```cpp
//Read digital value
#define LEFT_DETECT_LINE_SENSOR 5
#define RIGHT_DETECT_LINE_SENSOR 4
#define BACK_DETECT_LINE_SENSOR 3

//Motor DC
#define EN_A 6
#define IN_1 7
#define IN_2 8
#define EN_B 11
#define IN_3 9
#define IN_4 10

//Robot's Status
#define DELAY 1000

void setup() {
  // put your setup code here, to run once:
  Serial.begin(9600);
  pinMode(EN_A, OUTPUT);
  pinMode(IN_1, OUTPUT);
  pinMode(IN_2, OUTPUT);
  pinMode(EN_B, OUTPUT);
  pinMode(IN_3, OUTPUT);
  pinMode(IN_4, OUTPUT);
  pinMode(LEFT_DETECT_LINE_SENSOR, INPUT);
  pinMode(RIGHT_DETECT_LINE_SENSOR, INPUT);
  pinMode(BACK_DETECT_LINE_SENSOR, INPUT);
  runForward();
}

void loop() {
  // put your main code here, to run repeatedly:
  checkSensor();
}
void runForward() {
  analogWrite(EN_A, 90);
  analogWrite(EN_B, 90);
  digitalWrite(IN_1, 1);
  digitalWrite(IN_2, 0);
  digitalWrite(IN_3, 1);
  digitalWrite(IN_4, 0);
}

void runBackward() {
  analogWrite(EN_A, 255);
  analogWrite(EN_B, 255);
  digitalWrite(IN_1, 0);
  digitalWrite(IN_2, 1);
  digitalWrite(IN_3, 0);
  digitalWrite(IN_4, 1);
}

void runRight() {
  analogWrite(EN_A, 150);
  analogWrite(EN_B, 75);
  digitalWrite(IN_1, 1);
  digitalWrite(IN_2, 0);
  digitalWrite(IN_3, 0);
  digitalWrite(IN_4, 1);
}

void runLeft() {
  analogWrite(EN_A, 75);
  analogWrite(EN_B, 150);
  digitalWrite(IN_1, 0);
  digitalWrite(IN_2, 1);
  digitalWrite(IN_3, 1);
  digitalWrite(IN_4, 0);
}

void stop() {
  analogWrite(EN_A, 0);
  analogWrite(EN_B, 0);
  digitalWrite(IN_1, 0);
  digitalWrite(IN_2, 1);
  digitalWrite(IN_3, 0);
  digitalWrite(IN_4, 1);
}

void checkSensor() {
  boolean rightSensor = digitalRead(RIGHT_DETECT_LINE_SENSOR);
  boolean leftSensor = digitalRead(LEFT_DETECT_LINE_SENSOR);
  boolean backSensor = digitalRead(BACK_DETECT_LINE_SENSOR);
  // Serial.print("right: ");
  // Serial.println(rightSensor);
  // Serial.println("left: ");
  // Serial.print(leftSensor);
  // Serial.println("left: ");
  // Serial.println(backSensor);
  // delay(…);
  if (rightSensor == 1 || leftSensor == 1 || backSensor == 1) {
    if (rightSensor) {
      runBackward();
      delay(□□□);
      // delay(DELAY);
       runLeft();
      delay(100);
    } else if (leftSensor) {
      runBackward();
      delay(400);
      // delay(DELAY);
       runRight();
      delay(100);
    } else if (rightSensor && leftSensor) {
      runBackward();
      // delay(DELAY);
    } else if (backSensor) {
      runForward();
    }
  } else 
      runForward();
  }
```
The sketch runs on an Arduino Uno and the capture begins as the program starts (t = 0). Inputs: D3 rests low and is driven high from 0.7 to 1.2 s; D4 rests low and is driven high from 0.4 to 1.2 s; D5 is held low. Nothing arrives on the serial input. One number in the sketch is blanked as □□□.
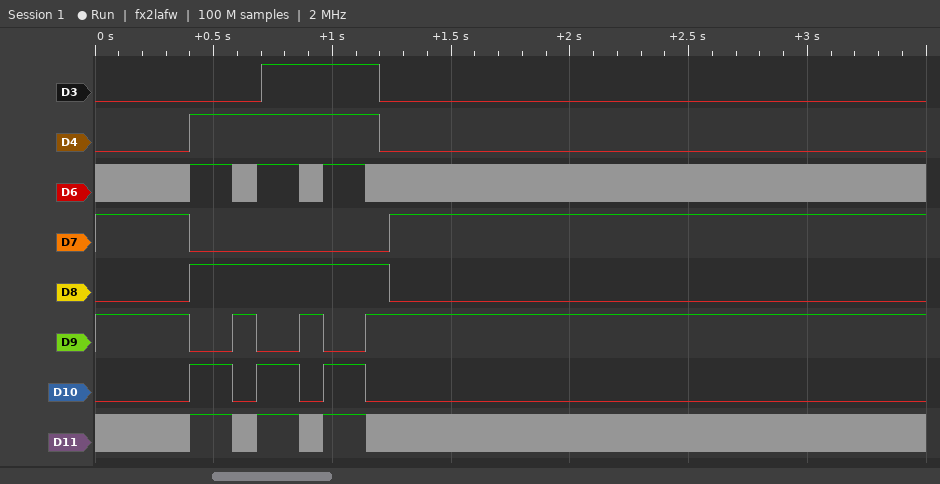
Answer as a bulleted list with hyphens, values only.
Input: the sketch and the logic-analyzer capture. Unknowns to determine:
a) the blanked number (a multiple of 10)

- 180
